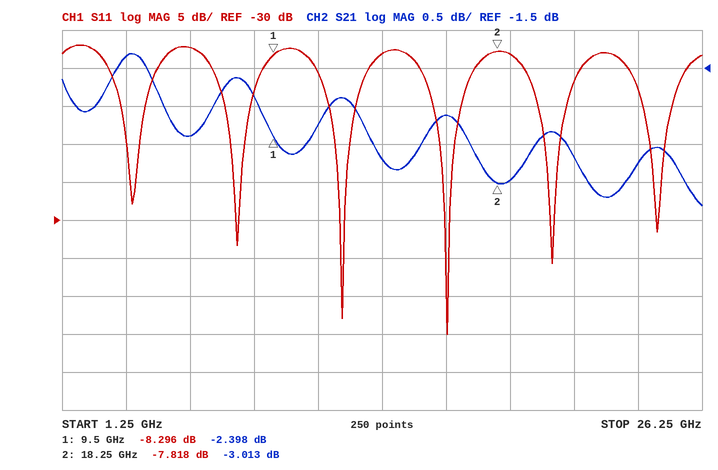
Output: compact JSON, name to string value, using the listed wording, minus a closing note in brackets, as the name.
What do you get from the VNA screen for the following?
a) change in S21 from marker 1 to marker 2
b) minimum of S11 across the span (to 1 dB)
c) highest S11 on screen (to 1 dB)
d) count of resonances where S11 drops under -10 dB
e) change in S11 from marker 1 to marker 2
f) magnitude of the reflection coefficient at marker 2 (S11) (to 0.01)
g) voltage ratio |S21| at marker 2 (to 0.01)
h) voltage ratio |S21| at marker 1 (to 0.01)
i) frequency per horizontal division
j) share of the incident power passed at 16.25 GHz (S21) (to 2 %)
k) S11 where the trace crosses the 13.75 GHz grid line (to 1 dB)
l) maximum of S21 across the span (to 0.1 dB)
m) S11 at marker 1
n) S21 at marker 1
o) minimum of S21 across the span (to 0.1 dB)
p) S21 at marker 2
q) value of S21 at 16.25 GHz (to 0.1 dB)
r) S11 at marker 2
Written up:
{"change in S21 from marker 1 to marker 2": "-0.615 dB", "minimum of S11 across the span": "-45 dB", "highest S11 on screen": "-7 dB", "count of resonances where S11 drops under -10 dB": "6", "change in S11 from marker 1 to marker 2": "0.478 dB", "magnitude of the reflection coefficient at marker 2 (S11)": "0.41", "voltage ratio |S21| at marker 2": "0.71", "voltage ratio |S21| at marker 1": "0.76", "frequency per horizontal division": "2.5 GHz", "share of the incident power passed at 16.25 GHz (S21)": "62 %", "S11 where the trace crosses the 13.75 GHz grid line": "-8 dB", "maximum of S21 across the span": "-1.3 dB", "S11 at marker 1": "-8.296 dB", "S21 at marker 1": "-2.398 dB", "minimum of S21 across the span": "-3.3 dB", "S21 at marker 2": "-3.013 dB", "value of S21 at 16.25 GHz": "-2.1 dB", "S11 at marker 2": "-7.818 dB"}
